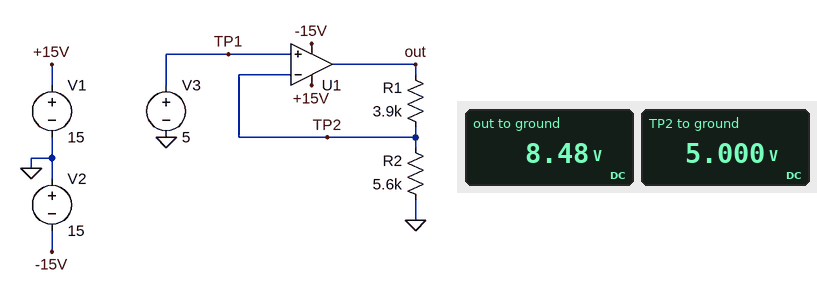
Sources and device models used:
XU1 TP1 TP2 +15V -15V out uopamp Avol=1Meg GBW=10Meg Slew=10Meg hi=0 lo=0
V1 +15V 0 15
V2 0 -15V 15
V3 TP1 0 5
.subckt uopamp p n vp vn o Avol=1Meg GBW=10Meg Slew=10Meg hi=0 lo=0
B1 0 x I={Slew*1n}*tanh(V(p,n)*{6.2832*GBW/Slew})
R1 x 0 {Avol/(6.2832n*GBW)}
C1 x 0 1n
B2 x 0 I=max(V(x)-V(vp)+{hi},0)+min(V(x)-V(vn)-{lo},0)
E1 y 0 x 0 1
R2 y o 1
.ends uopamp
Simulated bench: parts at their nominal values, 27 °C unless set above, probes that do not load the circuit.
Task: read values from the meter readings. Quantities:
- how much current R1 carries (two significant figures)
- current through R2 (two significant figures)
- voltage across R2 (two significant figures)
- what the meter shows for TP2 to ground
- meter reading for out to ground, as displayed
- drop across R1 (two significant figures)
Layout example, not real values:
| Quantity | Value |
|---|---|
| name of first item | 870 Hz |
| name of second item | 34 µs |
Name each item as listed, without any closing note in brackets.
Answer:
| Quantity | Value |
|---|---|
| how much current R1 carries | 890 µA |
| current through R2 | 890 µA |
| voltage across R2 | 5.0 V |
| what the meter shows for TP2 to ground | 5.000 V |
| meter reading for out to ground, as displayed | 8.48 V |
| drop across R1 | 3.5 V |
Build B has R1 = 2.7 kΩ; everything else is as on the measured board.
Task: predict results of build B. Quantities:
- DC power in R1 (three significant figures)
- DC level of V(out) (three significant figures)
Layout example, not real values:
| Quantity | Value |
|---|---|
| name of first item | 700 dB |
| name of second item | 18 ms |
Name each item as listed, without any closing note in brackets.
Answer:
| Quantity | Value |
|---|---|
| DC power in R1 | 2.15 mW |
| DC level of V(out) | 7.41 V |
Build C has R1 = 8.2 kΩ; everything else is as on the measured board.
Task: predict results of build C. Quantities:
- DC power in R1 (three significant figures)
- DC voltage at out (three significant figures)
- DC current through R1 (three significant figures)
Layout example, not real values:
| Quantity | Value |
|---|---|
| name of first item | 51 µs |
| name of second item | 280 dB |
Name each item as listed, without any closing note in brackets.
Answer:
| Quantity | Value |
|---|---|
| DC power in R1 | 6.54 mW |
| DC voltage at out | 12.3 V |
| DC current through R1 | 893 µA |
